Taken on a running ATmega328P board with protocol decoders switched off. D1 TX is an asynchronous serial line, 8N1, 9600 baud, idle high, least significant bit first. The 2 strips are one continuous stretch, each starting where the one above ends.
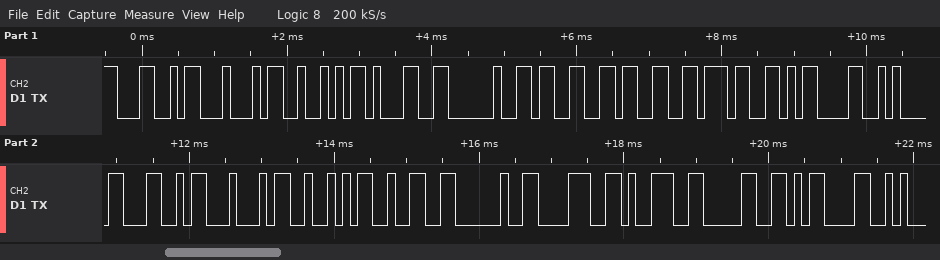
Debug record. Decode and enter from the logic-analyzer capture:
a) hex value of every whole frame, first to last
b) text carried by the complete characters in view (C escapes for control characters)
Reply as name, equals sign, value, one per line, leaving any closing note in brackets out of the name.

hex value of every whole frame, first to last = 4C 44 52 31 20 33 33 37 0D 0A 4C 44 52 32 20 38 39 30 0D
text carried by the complete characters in view = "LDR1 337\r\nLDR2 890\r"
